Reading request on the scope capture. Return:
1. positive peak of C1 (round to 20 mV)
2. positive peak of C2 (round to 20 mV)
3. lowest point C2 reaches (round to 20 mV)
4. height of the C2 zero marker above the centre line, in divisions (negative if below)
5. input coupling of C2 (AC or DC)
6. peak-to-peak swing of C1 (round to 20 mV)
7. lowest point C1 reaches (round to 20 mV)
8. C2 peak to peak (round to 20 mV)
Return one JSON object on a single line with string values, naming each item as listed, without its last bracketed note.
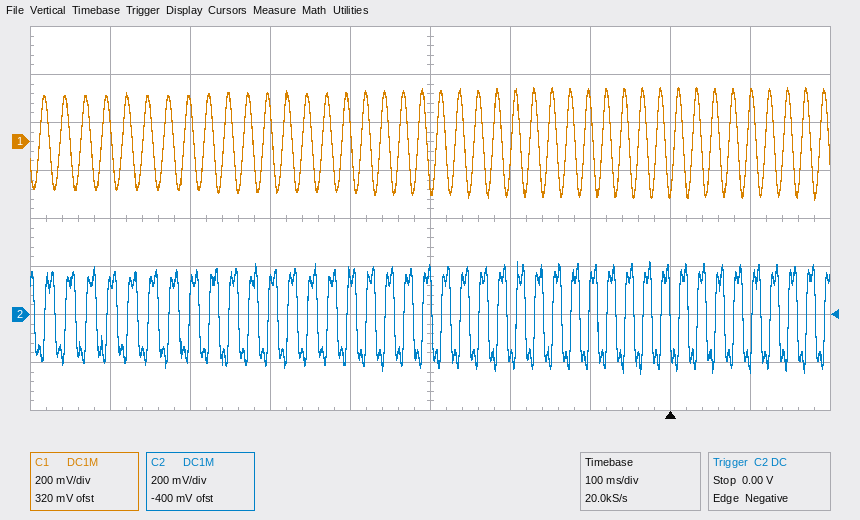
{"positive peak of C1": "220 mV", "positive peak of C2": "220 mV", "lowest point C2 reaches": "-240 mV", "height of the C2 zero marker above the centre line, in divisions": "-2.0 div", "input coupling of C2": "DC", "peak-to-peak swing of C1": "460 mV", "lowest point C1 reaches": "-240 mV", "C2 peak to peak": "460 mV"}
